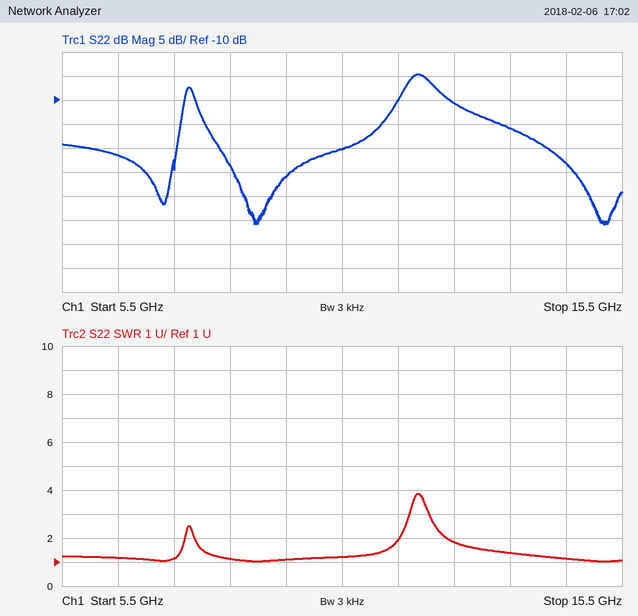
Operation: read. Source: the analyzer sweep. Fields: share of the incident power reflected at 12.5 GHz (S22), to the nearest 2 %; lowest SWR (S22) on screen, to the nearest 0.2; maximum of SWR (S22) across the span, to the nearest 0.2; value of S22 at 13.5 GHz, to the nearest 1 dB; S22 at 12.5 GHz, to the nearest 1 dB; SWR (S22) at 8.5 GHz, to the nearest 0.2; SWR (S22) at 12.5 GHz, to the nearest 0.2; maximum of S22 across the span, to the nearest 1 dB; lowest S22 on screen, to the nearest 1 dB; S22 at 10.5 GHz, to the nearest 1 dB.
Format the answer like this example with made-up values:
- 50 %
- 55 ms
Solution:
- 8 %
- 1.0
- 3.8
- -16 dB
- -11 dB
- 1.2
- 1.8
- -5 dB
- -36 dB
- -20 dB
